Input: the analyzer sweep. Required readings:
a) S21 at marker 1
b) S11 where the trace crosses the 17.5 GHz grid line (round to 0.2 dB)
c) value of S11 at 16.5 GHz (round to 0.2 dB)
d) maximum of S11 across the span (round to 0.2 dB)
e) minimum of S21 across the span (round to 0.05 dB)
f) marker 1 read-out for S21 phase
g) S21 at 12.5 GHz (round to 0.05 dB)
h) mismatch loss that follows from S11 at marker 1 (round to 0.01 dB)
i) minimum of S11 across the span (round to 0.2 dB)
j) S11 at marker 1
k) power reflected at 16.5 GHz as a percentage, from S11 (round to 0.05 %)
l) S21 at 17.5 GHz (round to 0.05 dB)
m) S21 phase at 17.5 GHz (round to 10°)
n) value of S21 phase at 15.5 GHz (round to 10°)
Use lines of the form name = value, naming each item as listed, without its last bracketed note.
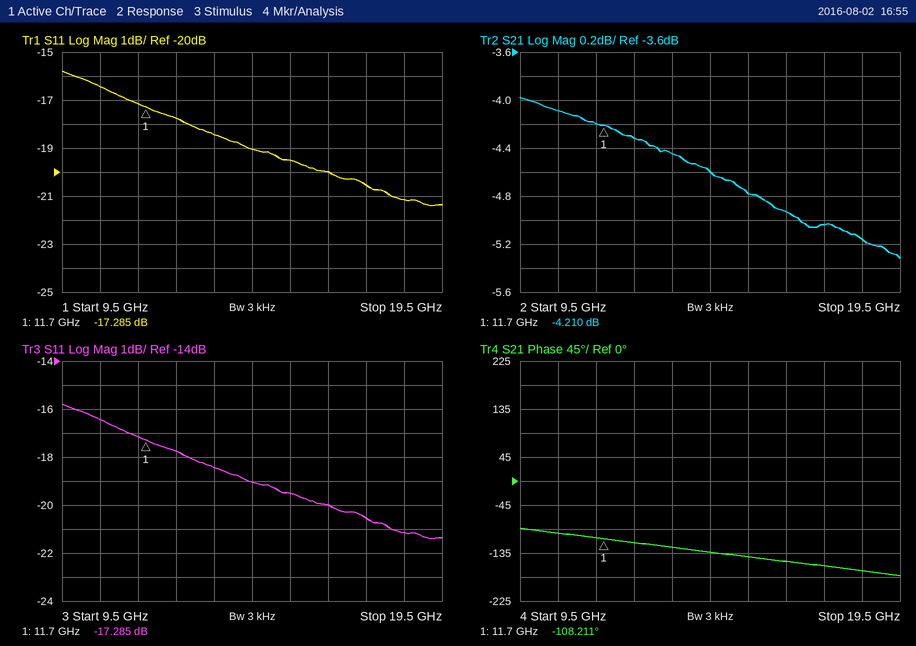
S21 at marker 1 = -4.210 dB
S11 where the trace crosses the 17.5 GHz grid line = -20.6 dB
value of S11 at 16.5 GHz = -20.0 dB
maximum of S11 across the span = -15.8 dB
minimum of S21 across the span = -5.30 dB
marker 1 read-out for S21 phase = -108.211°
S21 at 12.5 GHz = -4.30 dB
mismatch loss that follows from S11 at marker 1 = 0.08 dB
minimum of S11 across the span = -21.4 dB
S11 at marker 1 = -17.285 dB
power reflected at 16.5 GHz as a percentage, from S11 = 1.00 %
S21 at 17.5 GHz = -5.05 dB
S21 phase at 17.5 GHz = -160°
value of S21 phase at 15.5 GHz = -140°
